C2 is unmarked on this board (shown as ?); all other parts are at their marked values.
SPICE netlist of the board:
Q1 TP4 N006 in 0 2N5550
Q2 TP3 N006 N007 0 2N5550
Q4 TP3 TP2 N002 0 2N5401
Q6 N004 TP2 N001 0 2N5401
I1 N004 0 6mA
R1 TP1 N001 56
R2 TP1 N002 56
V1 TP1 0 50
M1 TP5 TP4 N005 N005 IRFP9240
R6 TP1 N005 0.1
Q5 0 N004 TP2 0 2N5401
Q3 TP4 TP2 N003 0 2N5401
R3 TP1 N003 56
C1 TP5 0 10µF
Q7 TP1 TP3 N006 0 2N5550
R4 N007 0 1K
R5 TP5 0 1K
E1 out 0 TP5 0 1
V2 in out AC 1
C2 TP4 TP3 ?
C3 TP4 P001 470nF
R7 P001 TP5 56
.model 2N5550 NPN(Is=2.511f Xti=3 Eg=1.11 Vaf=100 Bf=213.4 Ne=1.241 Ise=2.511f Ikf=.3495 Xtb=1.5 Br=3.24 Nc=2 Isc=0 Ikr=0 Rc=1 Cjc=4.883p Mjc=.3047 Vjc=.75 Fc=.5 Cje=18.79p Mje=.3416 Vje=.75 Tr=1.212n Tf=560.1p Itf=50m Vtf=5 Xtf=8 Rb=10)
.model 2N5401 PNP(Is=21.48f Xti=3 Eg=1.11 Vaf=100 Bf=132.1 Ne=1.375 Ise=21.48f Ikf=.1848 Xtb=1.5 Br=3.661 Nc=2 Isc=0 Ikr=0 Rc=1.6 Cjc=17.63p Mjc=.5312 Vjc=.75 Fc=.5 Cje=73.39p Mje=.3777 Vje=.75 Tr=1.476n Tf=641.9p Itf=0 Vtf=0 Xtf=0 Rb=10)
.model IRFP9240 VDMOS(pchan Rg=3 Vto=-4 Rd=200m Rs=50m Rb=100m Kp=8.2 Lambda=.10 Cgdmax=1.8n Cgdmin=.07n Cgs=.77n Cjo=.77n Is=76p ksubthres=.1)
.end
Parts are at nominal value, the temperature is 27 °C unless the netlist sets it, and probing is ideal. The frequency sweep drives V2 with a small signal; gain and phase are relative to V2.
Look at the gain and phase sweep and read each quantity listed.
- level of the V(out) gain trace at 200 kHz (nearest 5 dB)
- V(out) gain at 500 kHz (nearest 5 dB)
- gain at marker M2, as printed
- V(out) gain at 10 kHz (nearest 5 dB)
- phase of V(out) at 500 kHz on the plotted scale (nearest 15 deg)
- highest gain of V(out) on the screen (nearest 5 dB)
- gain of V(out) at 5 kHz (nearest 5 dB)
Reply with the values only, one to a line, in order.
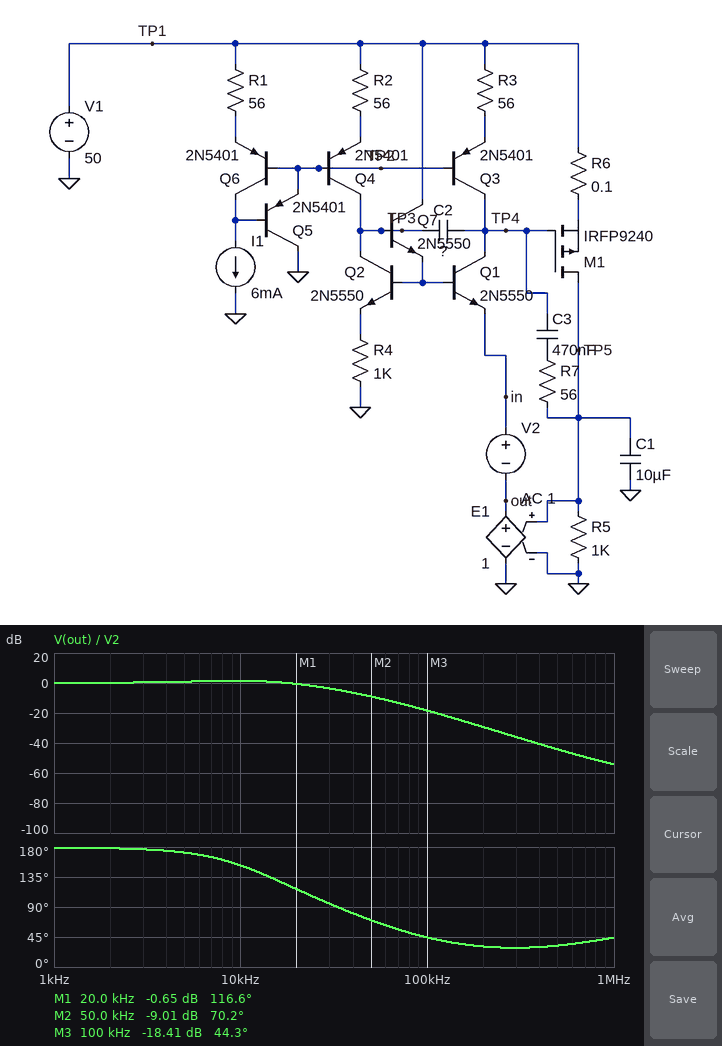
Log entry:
-30 dB
-45 dB
-9.01 dB
0 dB
30 deg
0 dB
0 dB
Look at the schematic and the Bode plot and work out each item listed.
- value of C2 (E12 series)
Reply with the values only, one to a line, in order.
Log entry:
150 pF
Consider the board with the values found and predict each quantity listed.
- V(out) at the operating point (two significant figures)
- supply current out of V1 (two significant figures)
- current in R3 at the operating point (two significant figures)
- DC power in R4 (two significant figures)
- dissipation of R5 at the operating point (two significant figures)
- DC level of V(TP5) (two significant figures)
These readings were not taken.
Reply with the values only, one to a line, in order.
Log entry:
6.2 V
25 mA
6.1 mA
39 mW
39 mW
6.2 V
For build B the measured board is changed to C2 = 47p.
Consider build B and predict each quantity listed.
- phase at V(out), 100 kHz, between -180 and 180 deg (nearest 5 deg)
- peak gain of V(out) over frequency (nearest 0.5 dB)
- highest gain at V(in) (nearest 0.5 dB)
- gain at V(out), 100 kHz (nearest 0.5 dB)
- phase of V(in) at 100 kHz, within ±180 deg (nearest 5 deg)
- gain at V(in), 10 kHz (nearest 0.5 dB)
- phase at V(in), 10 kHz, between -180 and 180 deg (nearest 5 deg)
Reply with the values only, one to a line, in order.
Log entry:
75 deg
1.0 dB
0.5 dB
-15.0 dB
10 deg
-6.0 dB
90 deg
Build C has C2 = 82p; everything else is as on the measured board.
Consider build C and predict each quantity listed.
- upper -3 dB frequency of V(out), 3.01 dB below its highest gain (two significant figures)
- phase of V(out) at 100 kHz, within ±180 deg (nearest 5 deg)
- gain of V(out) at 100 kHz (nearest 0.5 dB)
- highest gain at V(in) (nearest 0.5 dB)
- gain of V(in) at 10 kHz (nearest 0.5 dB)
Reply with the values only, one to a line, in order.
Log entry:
22 kHz
60 deg
-16.0 dB
1.0 dB
-5.5 dB
